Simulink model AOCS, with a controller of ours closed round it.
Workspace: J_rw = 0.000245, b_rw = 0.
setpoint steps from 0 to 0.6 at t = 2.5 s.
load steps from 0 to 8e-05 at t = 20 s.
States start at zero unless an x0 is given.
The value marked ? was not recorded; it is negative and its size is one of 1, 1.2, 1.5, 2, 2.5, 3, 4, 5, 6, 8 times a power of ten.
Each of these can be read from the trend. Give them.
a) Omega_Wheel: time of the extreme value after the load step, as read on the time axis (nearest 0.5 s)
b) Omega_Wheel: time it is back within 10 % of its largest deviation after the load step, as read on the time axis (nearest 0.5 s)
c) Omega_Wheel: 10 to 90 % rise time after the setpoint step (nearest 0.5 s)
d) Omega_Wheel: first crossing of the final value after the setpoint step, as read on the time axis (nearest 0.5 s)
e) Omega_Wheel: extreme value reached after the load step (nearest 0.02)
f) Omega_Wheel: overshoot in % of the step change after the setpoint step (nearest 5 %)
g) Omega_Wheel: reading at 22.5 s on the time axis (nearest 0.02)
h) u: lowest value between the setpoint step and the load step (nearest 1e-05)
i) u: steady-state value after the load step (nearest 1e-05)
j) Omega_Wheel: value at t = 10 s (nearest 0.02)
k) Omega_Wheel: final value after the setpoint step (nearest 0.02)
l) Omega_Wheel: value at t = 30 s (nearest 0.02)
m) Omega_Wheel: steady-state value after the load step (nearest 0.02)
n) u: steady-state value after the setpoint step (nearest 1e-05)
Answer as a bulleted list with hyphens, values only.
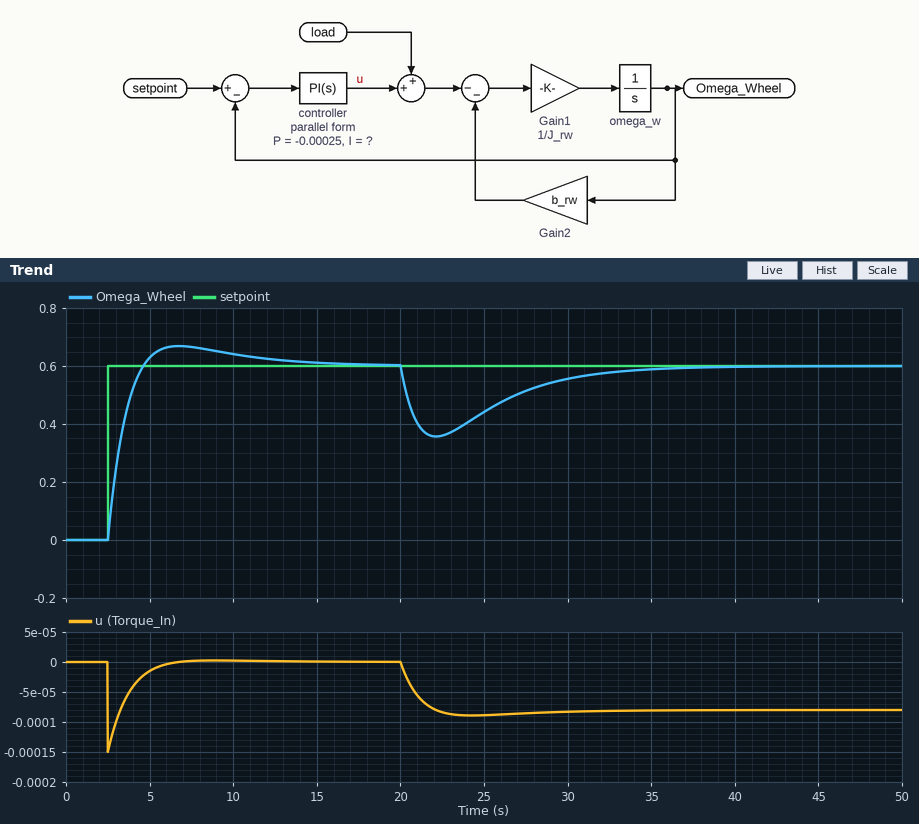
- 22.0 s
- 32.0 s
- 1.5 s
- 4.5 s
- 0.36
- 10 %
- 0.36
- -0.00015
- -0.00008
- 0.64
- 0.60
- 0.56
- 0.60
- 0.00000
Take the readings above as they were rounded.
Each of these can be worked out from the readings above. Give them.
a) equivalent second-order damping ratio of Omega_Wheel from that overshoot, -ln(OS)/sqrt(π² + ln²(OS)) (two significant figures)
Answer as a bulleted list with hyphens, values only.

- 0.59
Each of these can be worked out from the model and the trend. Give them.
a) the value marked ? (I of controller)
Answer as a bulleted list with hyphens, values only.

- -5e-05
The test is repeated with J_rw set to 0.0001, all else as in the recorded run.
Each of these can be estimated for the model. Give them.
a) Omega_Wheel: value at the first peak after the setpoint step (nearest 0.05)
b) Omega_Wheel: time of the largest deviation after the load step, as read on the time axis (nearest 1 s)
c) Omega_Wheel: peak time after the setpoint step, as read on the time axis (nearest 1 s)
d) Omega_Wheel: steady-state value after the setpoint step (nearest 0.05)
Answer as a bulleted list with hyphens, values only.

- 0.65
- 21 s
- 5 s
- 0.60
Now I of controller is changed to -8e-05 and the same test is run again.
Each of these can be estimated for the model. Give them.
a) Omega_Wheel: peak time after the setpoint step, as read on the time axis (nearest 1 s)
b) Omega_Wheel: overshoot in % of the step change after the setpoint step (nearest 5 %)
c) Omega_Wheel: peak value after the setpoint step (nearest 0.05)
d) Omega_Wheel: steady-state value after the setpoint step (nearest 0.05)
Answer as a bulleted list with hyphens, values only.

- 6 s
- 15 %
- 0.70
- 0.60
